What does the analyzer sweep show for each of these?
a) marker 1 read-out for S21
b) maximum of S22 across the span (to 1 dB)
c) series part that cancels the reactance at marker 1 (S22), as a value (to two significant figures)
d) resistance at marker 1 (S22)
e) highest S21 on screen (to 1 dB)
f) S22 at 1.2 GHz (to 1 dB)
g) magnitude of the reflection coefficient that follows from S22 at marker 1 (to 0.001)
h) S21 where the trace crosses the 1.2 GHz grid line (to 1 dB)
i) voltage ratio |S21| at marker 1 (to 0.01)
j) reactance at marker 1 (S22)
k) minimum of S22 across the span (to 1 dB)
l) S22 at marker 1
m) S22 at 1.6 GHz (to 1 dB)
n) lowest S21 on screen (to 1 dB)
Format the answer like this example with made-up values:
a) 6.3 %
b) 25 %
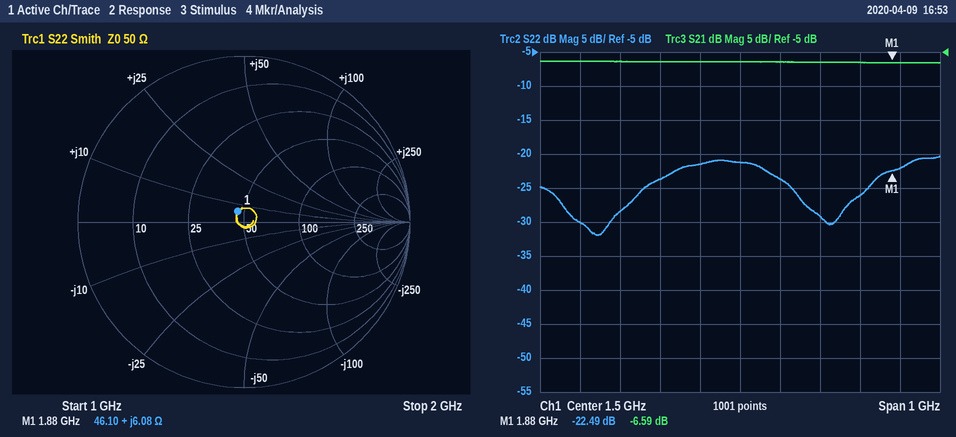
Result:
a) -6.59 dB
b) -20 dB
c) 14 pF
d) 46.10 Ω
e) -6 dB
f) -28 dB
g) 0.075
h) -6 dB
i) 0.47
j) +6.08 Ω
k) -32 dB
l) -22.49 dB
m) -24 dB
n) -7 dB
